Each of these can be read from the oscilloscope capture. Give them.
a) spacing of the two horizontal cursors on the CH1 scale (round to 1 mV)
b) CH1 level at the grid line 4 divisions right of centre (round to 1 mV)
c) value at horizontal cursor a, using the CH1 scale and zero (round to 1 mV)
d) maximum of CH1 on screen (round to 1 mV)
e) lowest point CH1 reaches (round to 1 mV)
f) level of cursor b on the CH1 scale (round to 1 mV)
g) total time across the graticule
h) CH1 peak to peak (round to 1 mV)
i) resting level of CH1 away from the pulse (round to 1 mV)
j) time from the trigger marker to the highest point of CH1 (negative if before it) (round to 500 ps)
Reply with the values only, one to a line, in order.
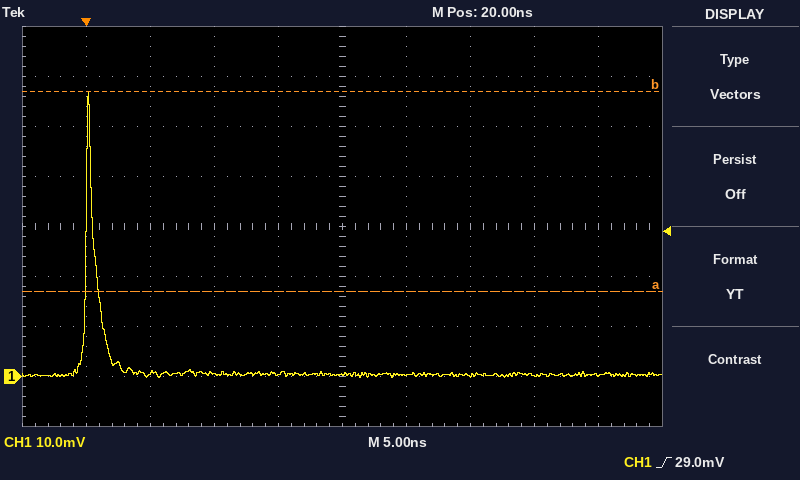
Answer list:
40 mV
0 mV
17 mV
57 mV
0 mV
57 mV
50 ns
57 mV
0 mV
0.0 ns
